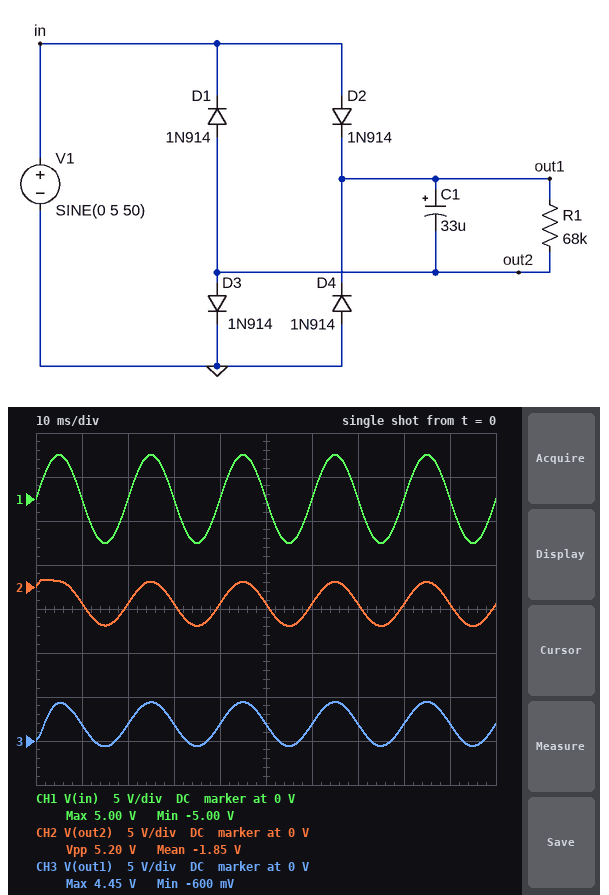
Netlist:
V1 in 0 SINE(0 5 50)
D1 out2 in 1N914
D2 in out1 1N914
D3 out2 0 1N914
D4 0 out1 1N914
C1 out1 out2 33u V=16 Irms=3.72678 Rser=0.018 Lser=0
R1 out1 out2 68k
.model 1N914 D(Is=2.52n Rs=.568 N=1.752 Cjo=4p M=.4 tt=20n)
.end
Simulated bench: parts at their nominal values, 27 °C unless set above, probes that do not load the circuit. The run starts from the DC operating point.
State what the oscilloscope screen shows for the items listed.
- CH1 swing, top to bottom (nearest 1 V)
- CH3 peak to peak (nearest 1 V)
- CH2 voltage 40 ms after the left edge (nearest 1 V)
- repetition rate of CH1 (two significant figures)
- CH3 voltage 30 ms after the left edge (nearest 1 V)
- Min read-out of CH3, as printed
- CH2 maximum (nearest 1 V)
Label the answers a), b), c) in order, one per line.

a) 10 V
b) 5 V
c) -2 V
d) 50 Hz
e) 2 V
f) -600 mV
g) 1 V
